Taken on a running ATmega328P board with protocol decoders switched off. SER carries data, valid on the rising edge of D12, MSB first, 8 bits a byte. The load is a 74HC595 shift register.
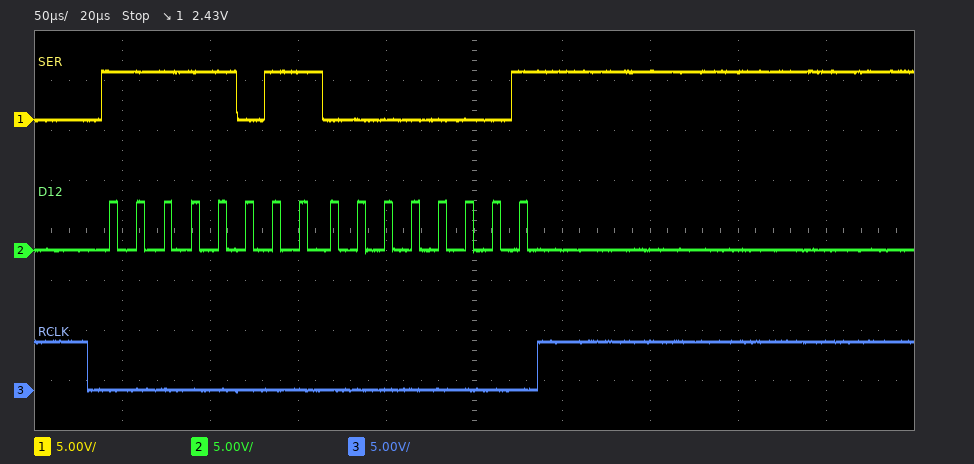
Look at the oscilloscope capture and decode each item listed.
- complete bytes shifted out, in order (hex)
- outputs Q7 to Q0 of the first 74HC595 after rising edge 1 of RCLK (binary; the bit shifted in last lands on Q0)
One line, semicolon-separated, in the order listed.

0xFB 0x01; 00000001
